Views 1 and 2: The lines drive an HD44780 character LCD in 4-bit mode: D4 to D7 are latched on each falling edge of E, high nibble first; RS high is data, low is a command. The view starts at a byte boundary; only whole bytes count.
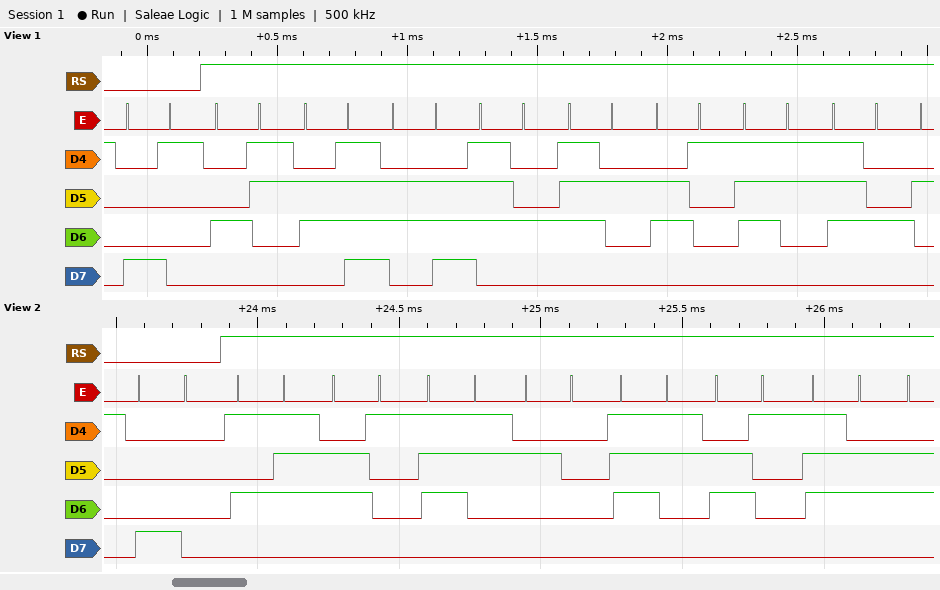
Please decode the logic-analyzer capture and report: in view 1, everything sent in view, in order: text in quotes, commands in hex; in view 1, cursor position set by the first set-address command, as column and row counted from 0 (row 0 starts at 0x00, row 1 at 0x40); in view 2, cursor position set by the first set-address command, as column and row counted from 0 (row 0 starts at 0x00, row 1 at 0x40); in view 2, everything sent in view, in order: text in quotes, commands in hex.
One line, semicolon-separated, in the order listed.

0x81 "Contrast"; column 1, row 0; column 0, row 0; 0x80 "Was sav"
